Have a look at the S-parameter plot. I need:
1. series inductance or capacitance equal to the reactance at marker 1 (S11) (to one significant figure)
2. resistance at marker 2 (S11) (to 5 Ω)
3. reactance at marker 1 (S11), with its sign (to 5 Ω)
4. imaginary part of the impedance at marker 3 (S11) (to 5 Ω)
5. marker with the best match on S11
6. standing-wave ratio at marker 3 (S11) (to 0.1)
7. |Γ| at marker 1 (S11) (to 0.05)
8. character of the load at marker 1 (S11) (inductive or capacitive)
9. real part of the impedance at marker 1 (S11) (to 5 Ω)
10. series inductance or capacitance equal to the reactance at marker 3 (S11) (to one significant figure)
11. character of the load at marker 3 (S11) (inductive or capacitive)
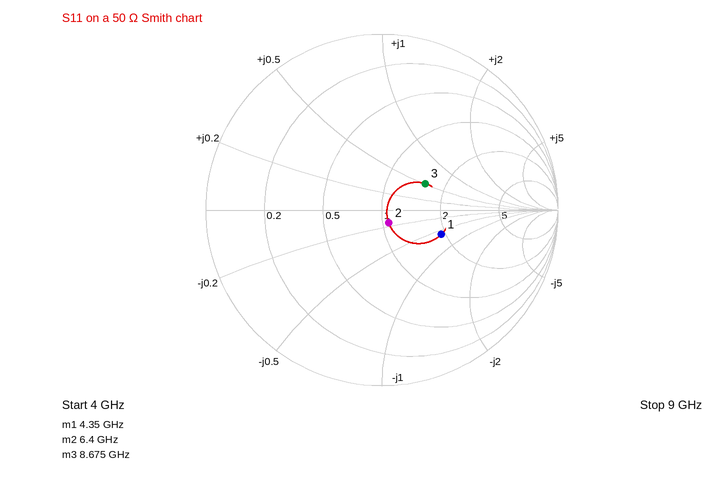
1 pF
55 Ω
-30 Ω
+25 Ω
marker 2
1.8
0.35
capacitive
95 Ω
500 pH
inductive
